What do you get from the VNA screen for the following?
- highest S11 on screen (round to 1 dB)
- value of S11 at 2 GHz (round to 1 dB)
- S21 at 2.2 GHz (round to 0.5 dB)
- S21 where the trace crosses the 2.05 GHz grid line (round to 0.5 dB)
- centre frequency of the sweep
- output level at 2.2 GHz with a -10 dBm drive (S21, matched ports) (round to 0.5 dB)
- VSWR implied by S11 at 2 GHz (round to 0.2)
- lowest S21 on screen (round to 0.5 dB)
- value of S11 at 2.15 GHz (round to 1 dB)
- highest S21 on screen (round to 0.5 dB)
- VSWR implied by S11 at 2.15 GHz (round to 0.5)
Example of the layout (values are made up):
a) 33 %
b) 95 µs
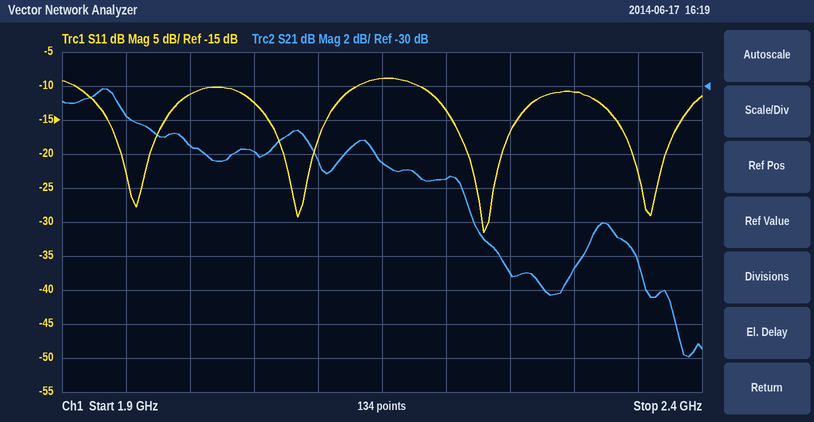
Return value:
a) -9 dB
b) -11 dB
c) -35.5 dB
d) -34.0 dB
e) 2.15 GHz
f) -45.5 dBm
g) 1.8
h) -46.0 dB
i) -9 dB
j) -30.0 dB
k) 2.0
